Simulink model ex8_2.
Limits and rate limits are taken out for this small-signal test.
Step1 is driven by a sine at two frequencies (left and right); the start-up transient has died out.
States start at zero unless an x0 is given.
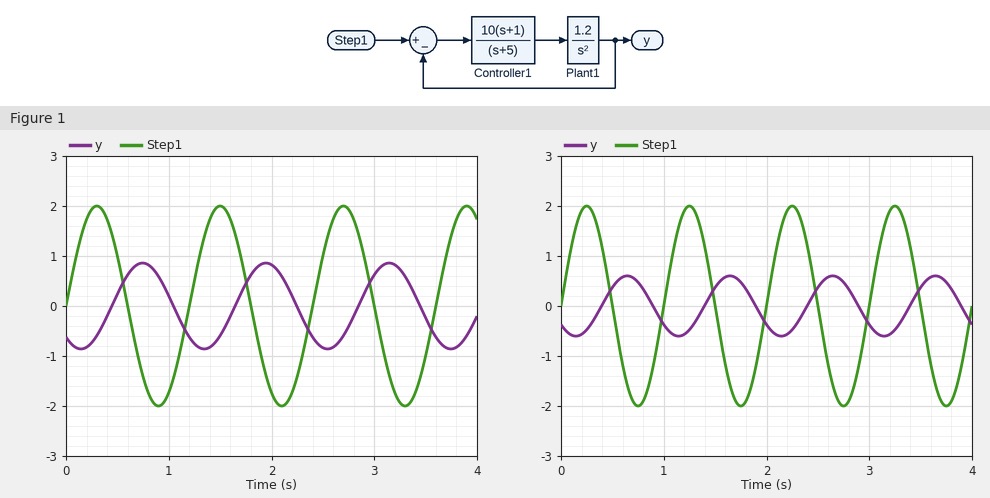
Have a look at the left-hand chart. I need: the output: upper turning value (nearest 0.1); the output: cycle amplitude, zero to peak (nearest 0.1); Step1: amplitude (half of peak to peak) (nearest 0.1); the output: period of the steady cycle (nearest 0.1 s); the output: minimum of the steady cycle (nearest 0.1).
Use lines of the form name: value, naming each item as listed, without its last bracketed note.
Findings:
the output: upper turning value: 0.9
the output: cycle amplitude, zero to peak: 0.9
Step1: amplitude (half of peak to peak): 2.0
the output: period of the steady cycle: 1.2 s
the output: minimum of the steady cycle: -0.9
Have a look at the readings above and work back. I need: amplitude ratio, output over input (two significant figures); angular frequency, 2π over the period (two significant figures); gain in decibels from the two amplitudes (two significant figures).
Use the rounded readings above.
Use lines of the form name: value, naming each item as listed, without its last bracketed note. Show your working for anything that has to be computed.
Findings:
amplitude ratio, output over input: 0.9 / 2 = 0.45
angular frequency, 2π over the period: 2π / 1.2 = 5.2 rad/s
gain in decibels from the two amplitudes: 20 log10(0.9 / 2) = -6.9 dB
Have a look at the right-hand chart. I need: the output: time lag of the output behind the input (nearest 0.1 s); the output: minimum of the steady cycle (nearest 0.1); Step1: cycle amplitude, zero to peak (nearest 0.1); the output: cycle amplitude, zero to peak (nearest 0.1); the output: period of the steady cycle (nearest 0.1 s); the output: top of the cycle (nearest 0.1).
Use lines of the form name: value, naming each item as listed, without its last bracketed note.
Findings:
the output: time lag of the output behind the input: 0.4 s
the output: minimum of the steady cycle: -0.6
Step1: cycle amplitude, zero to peak: 2.0
the output: cycle amplitude, zero to peak: 0.6
the output: period of the steady cycle: 1.0 s
the output: top of the cycle: 0.6
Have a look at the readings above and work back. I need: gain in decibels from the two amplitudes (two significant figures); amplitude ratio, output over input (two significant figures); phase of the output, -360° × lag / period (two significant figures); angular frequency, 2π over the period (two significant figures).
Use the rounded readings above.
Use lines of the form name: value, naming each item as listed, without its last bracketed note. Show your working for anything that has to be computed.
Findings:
gain in decibels from the two amplitudes: 20 log10(0.6 / 2) = -10 dB
amplitude ratio, output over input: 0.6 / 2 = 0.30
phase of the output, -360° × lag / period: -360 × 0.4 / 1 = -140°
angular frequency, 2π over the period: 2π / 1 = 6.3 rad/s
